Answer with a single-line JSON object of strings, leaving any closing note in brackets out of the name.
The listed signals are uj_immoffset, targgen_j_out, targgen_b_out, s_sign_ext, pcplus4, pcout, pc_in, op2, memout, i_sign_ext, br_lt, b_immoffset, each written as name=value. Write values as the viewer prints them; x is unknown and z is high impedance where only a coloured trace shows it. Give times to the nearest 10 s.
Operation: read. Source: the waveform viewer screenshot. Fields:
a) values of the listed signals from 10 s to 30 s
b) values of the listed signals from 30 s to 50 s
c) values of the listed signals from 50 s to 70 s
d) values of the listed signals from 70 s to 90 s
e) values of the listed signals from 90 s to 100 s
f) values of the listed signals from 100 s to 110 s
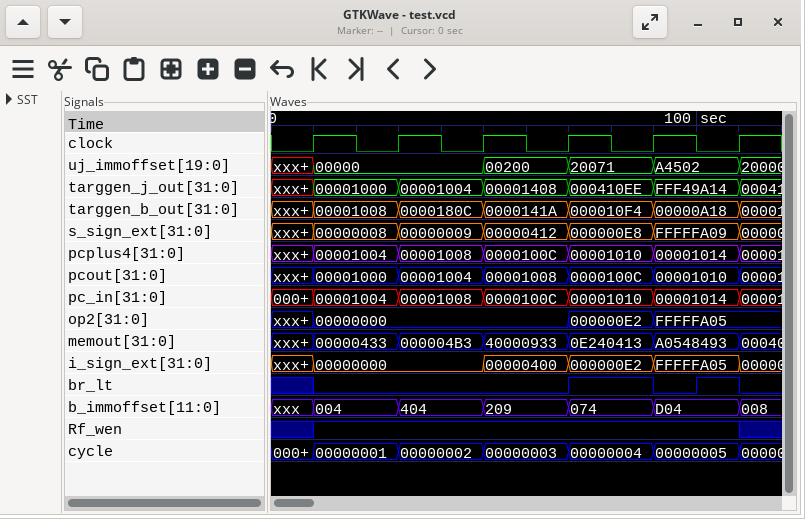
{"values of the listed signals from 10 s to 30 s": "uj_immoffset=00000, targgen_j_out=00001000, targgen_b_out=00001008, s_sign_ext=00000008, pcplus4=00001004, pcout=00001000, pc_in=00001004, op2=00000000, memout=00000433, i_sign_ext=00000000, br_lt=0, b_immoffset=004", "values of the listed signals from 30 s to 50 s": "uj_immoffset=00000, targgen_j_out=00001004, targgen_b_out=0000180C, s_sign_ext=00000009, pcplus4=00001008, pcout=00001004, pc_in=00001008, op2=00000000, memout=000004B3, i_sign_ext=00000000, br_lt=0, b_immoffset=404", "values of the listed signals from 50 s to 70 s": "uj_immoffset=00200, targgen_j_out=00001408, targgen_b_out=0000141A, s_sign_ext=00000412, pcplus4=0000100C, pcout=00001008, pc_in=0000100C, op2=00000000, memout=40000933, i_sign_ext=00000400, br_lt=0, b_immoffset=209", "values of the listed signals from 70 s to 90 s": "uj_immoffset=20071, targgen_j_out=000410EE, targgen_b_out=000010F4, s_sign_ext=000000E8, pcplus4=00001010, pcout=0000100C, pc_in=00001010, op2=000000E2, memout=0E240413, i_sign_ext=000000E2, br_lt=1, b_immoffset=074", "values of the listed signals from 90 s to 100 s": "uj_immoffset=A4502, targgen_j_out=FFF49A14, targgen_b_out=00000A18, s_sign_ext=FFFFFA09, pcplus4=00001014, pcout=00001010, pc_in=00001014, op2=FFFFFA05, memout=A0548493, i_sign_ext=FFFFFA05, br_lt=0, b_immoffset=D04", "values of the listed signals from 100 s to 110 s": "uj_immoffset=A4502, targgen_j_out=FFF49A14, targgen_b_out=00000A18, s_sign_ext=FFFFFA09, pcplus4=00001014, pcout=00001010, pc_in=00001014, op2=FFFFFA05, memout=A0548493, i_sign_ext=FFFFFA05, br_lt=1, b_immoffset=D04"}
